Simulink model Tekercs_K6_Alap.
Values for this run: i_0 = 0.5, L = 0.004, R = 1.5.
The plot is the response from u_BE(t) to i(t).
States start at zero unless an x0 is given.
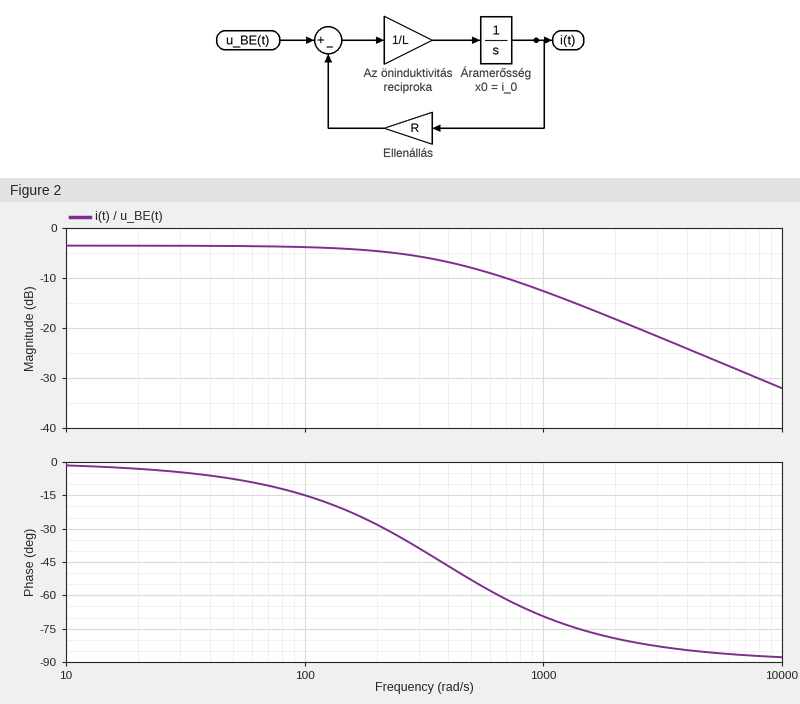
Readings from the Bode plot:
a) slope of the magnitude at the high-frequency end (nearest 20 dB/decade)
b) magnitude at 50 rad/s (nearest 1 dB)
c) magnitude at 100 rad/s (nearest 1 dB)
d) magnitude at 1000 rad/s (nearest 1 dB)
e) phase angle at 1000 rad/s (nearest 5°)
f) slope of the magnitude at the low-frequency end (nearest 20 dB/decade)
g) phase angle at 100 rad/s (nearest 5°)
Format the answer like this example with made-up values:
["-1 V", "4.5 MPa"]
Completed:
["-20 dB/decade", "-4 dB", "-4 dB", "-13 dB", "-70°", "0 dB/decade", "-15°"]
